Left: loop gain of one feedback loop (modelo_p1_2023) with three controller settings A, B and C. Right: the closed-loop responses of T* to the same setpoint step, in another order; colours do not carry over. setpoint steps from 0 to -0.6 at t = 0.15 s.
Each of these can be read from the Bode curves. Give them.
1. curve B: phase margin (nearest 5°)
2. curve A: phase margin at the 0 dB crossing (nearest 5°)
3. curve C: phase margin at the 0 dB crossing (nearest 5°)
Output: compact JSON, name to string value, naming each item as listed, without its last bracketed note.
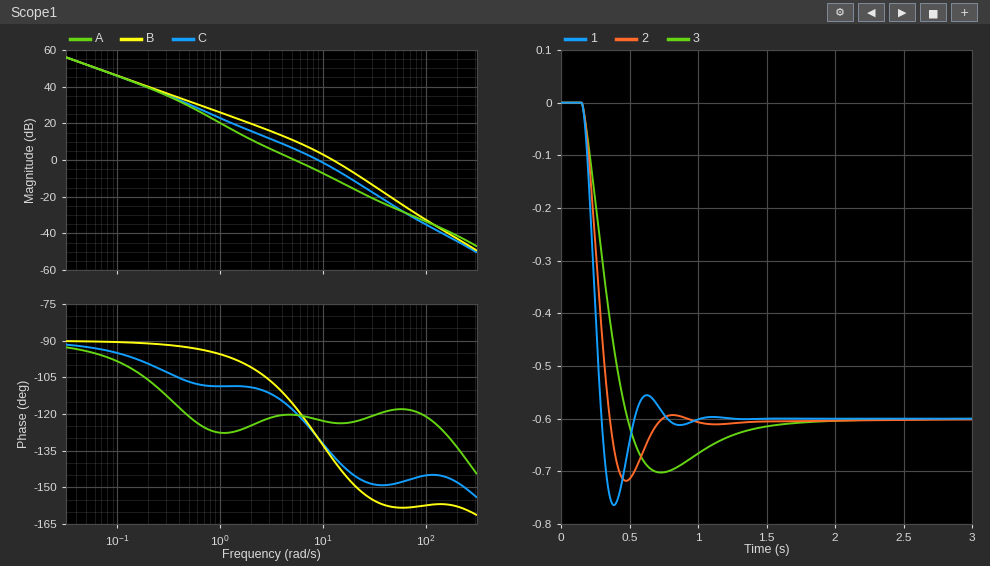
{"curve B: phase margin": "40°", "curve A: phase margin at the 0 dB crossing": "60°", "curve C: phase margin at the 0 dB crossing": "50°"}
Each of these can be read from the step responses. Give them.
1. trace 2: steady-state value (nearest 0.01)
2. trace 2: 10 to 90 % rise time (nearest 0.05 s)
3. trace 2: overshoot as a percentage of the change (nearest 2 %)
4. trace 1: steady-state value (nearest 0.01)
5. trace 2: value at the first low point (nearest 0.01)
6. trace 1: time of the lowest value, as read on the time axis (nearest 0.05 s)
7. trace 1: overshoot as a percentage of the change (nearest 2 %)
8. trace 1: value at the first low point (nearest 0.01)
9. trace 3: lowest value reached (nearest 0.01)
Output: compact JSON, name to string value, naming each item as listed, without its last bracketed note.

{"trace 2: steady-state value": "-0.60", "trace 2: 10 to 90 % rise time": "0.15 s", "trace 2: overshoot as a percentage of the change": "20 %", "trace 1: steady-state value": "-0.60", "trace 2: value at the first low point": "-0.72", "trace 1: time of the lowest value, as read on the time axis": "0.40 s", "trace 1: overshoot as a percentage of the change": "28 %", "trace 1: value at the first low point": "-0.76", "trace 3: lowest value reached": "-0.70"}
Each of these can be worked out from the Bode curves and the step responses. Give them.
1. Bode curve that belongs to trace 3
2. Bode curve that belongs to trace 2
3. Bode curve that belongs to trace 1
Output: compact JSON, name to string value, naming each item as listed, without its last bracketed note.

{"Bode curve that belongs to trace 3": "A", "Bode curve that belongs to trace 2": "C", "Bode curve that belongs to trace 1": "B"}
